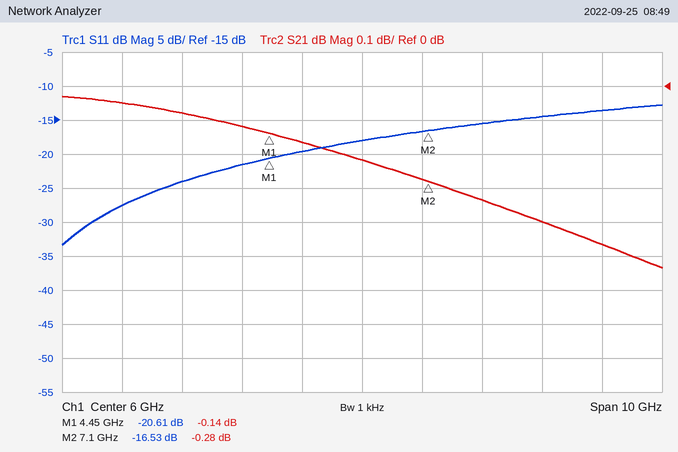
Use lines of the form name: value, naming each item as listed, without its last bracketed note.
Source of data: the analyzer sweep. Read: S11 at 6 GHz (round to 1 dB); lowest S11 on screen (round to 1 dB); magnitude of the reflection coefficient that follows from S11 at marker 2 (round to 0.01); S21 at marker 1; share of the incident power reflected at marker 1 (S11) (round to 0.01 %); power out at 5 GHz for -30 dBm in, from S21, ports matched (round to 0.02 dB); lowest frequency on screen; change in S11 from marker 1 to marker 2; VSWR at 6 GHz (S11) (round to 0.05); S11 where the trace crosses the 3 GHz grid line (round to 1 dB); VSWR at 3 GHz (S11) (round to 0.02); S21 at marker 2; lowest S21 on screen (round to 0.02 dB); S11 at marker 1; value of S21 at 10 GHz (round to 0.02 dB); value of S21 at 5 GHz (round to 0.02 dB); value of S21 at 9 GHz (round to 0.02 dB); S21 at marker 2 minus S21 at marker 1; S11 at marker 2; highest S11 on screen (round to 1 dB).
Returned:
S11 at 6 GHz: -18 dB
lowest S11 on screen: -33 dB
magnitude of the reflection coefficient that follows from S11 at marker 2: 0.15
S21 at marker 1: -0.14 dB
share of the incident power reflected at marker 1 (S11): 0.87 %
power out at 5 GHz for -30 dBm in, from S21, ports matched: -30.16 dBm
lowest frequency on screen: 1 GHz
change in S11 from marker 1 to marker 2: 4.08 dB
VSWR at 6 GHz (S11): 1.30
S11 where the trace crosses the 3 GHz grid line: -24 dB
VSWR at 3 GHz (S11): 1.14
S21 at marker 2: -0.28 dB
lowest S21 on screen: -0.54 dB
S11 at marker 1: -20.61 dB
value of S21 at 10 GHz: -0.46 dB
value of S21 at 5 GHz: -0.16 dB
value of S21 at 9 GHz: -0.40 dB
S21 at marker 2 minus S21 at marker 1: -0.14 dB
S11 at marker 2: -16.53 dB
highest S11 on screen: -13 dB
